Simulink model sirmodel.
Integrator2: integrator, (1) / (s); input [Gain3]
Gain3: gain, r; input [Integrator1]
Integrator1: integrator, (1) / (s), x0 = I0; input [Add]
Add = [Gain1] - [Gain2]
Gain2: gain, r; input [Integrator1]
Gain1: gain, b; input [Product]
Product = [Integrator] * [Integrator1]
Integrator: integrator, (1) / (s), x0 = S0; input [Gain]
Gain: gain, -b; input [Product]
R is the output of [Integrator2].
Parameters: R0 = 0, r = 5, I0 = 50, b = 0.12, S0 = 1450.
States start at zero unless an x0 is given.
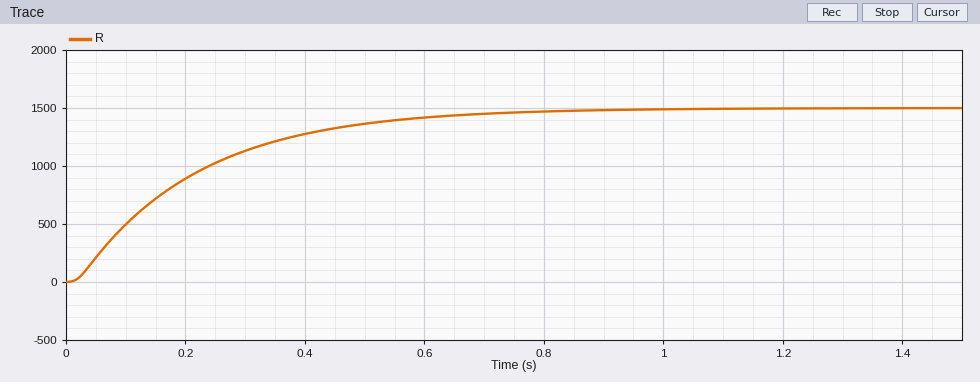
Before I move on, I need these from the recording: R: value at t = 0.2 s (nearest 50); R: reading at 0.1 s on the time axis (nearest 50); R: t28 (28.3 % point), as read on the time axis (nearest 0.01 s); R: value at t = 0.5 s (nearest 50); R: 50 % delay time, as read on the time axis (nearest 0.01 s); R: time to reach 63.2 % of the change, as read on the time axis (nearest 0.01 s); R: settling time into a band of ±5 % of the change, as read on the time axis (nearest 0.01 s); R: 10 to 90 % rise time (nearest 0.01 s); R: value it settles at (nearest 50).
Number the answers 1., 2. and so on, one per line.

1. 900
2. 500
3. 0.09 s
4. 1350
5. 0.16 s
6. 0.22 s
7. 0.62 s
8. 0.44 s
9. 1500
